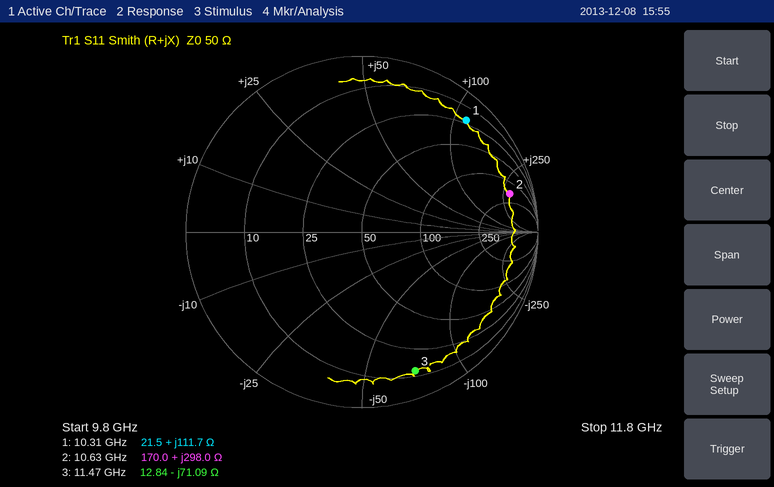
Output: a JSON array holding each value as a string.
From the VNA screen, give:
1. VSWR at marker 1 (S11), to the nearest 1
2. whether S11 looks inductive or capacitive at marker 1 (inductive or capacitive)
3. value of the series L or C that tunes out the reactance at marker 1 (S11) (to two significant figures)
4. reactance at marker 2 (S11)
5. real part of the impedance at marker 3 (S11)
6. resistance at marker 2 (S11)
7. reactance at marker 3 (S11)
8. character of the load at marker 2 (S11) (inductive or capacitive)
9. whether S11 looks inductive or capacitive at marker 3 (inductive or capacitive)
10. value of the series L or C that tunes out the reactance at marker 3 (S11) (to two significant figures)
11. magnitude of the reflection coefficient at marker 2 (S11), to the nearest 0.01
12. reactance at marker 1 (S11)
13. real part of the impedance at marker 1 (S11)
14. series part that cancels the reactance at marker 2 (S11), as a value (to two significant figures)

["14", "inductive", "140 fF", "+298.0 Ω", "12.84 Ω", "170.0 Ω", "-71.09 Ω", "inductive", "capacitive", "990 pH", "0.87", "+111.7 Ω", "21.5 Ω", "50 fF"]
